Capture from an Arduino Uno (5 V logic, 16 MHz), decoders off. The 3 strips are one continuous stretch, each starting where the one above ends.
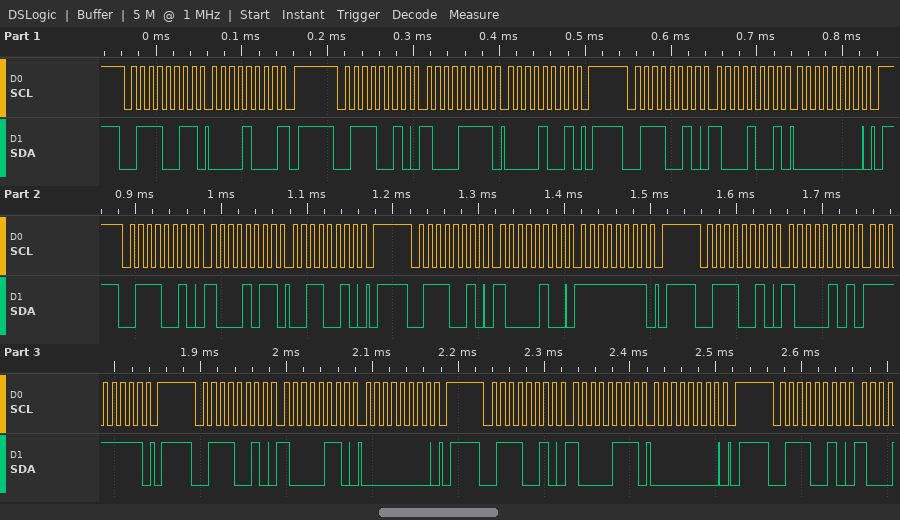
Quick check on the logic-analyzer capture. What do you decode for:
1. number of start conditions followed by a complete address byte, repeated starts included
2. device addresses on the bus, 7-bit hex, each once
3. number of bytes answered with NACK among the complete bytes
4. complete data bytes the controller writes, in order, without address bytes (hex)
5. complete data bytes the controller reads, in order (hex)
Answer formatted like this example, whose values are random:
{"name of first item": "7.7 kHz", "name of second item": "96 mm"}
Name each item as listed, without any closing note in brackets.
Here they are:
{"number of start conditions followed by a complete address byte, repeated starts included": "9", "device addresses on the bus, 7-bit hex, each once": "0x39", "number of bytes answered with NACK among the complete bytes": "1", "complete data bytes the controller writes, in order, without address bytes": "8F 09 89 00 8B 32 84 FF 85 FF 86 00 87 00", "complete data bytes the controller reads, in order": "08"}
